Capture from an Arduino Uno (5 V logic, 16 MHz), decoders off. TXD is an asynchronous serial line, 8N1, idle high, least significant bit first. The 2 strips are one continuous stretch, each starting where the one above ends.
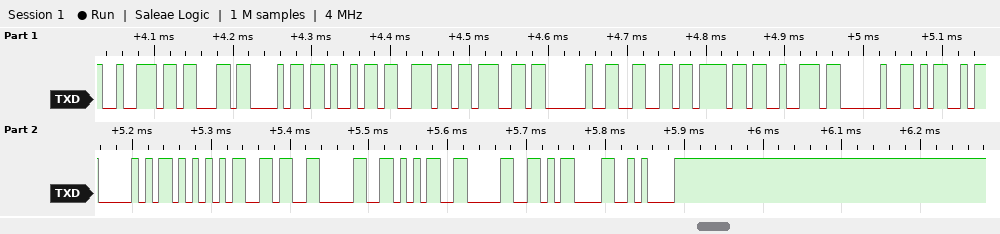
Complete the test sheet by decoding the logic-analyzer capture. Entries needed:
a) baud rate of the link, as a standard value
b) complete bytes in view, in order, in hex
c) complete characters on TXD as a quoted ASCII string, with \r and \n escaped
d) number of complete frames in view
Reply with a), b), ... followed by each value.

a) 115200 baud
b) 0x72 0x63 0x68 0x69 0x6E 0x67 0x20 0x66 0x6F 0x72 0x20 0x4D 0x50 0x55 0x36 0x30 0x35 0x30 0x0D 0x0A
c) "rching for MPU6050\r\n"
d) 20
